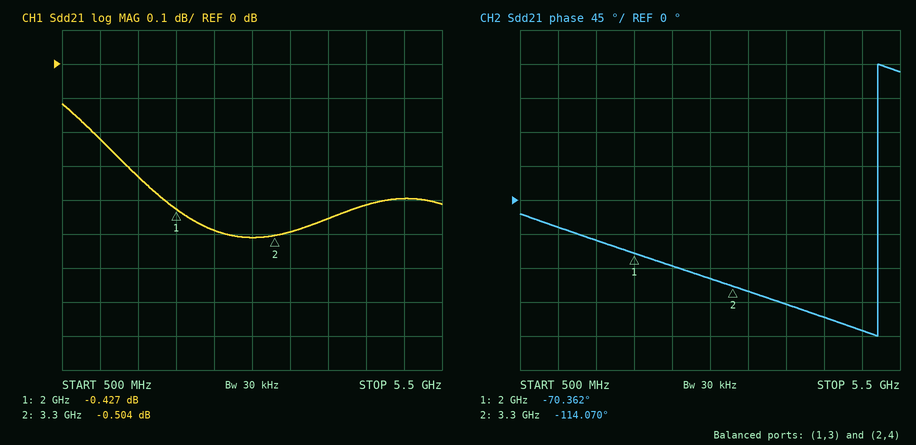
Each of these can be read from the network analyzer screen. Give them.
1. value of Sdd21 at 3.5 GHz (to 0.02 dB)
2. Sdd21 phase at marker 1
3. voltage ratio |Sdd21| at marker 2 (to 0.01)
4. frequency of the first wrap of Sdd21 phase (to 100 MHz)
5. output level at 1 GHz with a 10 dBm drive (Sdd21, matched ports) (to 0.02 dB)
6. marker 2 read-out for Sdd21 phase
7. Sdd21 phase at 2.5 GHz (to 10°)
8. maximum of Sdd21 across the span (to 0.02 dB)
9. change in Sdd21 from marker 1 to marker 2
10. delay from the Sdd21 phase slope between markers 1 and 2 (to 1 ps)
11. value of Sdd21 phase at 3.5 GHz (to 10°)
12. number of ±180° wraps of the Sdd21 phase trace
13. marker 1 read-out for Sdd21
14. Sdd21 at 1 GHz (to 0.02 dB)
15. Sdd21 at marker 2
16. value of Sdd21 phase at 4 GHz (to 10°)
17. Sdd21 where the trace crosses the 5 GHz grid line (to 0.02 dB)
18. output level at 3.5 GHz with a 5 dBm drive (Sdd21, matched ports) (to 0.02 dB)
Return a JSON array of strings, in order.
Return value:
["-0.50 dB", "-70.362°", "0.94", "5.2 GHz", "9.78 dBm", "-114.070°", "-90°", "-0.12 dB", "-0.077 dB", "93 ps", "-120°", "1", "-0.427 dB", "-0.22 dB", "-0.504 dB", "-140°", "-0.40 dB", "4.50 dBm"]
